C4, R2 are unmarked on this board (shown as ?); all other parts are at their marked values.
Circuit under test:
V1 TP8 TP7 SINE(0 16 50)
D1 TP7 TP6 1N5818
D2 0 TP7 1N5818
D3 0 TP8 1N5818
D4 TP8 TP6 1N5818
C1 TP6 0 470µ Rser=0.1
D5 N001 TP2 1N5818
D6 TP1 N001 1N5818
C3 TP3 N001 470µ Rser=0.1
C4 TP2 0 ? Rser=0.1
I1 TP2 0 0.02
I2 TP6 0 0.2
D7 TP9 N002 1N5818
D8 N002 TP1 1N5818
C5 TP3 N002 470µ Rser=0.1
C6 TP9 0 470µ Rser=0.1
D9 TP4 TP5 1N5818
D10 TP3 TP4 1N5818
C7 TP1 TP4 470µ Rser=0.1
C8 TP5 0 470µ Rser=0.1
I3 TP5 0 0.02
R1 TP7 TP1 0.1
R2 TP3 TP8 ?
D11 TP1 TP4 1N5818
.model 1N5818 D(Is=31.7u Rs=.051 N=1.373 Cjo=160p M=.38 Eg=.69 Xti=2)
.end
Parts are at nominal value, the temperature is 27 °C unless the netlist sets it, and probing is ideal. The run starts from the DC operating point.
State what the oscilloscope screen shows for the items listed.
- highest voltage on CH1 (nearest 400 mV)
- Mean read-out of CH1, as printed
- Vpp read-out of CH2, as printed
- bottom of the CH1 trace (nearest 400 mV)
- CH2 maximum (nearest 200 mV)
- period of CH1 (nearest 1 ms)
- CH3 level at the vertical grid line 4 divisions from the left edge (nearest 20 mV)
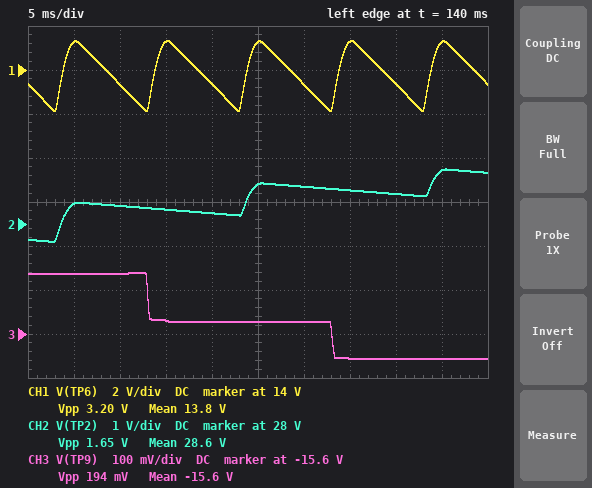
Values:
15.2 V
13.8 V
1.65 V
12.0 V
29.2 V
10 ms
-15.58 V
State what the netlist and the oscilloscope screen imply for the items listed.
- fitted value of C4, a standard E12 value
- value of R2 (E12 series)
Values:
1.2 mF
0.33 Ω
